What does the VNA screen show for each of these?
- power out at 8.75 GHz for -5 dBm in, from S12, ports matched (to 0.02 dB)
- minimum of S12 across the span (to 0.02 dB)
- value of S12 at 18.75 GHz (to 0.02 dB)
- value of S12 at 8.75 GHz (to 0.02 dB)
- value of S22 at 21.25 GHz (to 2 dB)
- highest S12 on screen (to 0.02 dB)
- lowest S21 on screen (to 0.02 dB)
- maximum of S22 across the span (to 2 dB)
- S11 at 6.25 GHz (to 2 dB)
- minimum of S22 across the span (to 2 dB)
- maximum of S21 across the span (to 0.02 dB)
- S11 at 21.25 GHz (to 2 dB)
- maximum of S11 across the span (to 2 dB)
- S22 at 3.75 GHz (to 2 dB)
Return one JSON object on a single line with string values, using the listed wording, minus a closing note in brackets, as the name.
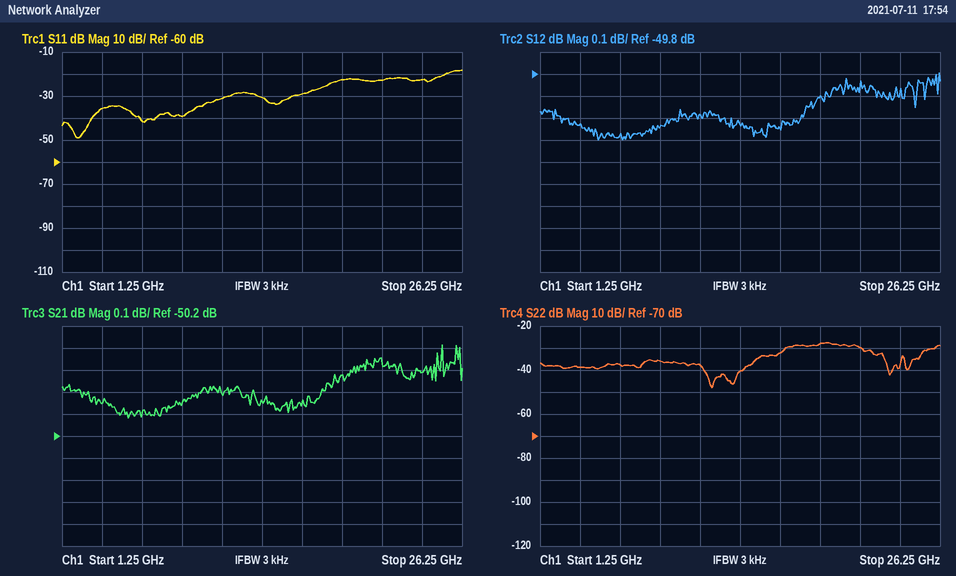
{"power out at 8.75 GHz for -5 dBm in, from S12, ports matched": "-55.04 dBm", "minimum of S12 across the span": "-50.10 dB", "value of S12 at 18.75 GHz": "-49.90 dB", "value of S12 at 8.75 GHz": "-50.04 dB", "value of S22 at 21.25 GHz": "-30 dB", "highest S12 on screen": "-49.80 dB", "lowest S21 on screen": "-50.12 dB", "maximum of S22 across the span": "-28 dB", "S11 at 6.25 GHz": "-42 dB", "minimum of S22 across the span": "-48 dB", "maximum of S21 across the span": "-49.78 dB", "S11 at 21.25 GHz": "-22 dB", "maximum of S11 across the span": "-18 dB", "S22 at 3.75 GHz": "-38 dB"}
